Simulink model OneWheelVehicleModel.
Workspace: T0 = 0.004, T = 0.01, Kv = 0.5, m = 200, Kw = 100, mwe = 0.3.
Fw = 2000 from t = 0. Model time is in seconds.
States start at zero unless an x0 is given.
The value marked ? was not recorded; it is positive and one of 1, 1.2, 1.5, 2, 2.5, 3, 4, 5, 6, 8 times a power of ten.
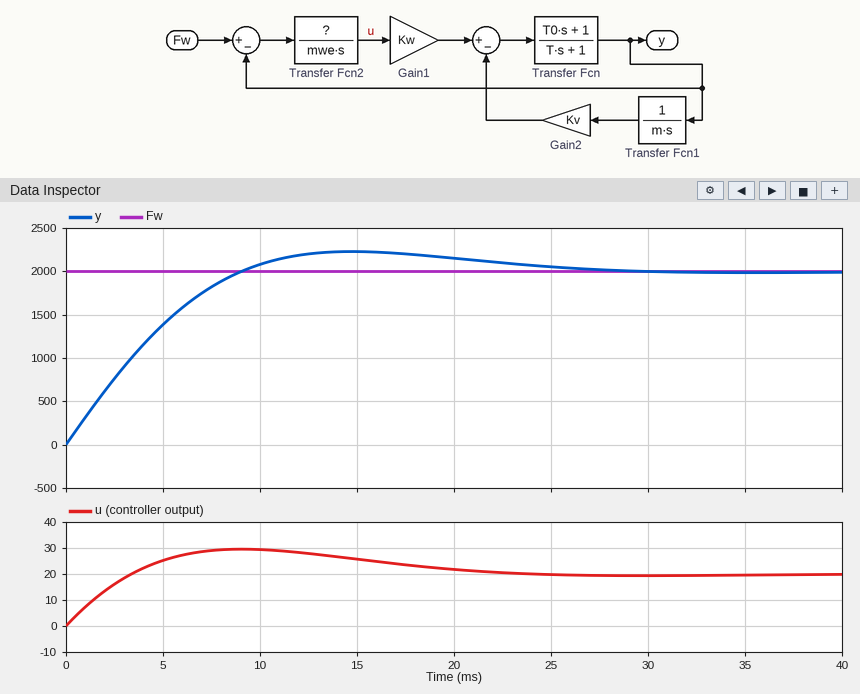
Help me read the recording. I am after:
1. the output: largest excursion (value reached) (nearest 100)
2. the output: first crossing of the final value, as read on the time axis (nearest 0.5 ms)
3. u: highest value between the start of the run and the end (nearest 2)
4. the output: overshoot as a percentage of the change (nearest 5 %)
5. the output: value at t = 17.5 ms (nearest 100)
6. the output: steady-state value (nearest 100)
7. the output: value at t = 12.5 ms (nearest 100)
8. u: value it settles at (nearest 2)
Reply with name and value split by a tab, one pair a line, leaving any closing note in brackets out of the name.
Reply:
the output: largest excursion (value reached)	2200
the output: first crossing of the final value, as read on the time axis	9.0 ms
u: highest value between the start of the run and the end	30
the output: overshoot as a percentage of the change	10 %
the output: value at t = 17.5 ms	2200
the output: steady-state value	2000
the output: value at t = 12.5 ms	2200
u: value it settles at	20
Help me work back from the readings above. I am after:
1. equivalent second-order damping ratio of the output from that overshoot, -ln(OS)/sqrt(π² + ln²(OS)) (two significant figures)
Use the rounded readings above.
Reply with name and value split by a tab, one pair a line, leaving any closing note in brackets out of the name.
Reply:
equivalent second-order damping ratio of the output from that overshoot, -ln(OS)/sqrt(π² + ln²(OS))	0.59
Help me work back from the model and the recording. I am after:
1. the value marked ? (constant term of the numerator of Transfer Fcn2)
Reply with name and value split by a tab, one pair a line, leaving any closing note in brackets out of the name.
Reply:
the value marked ?	1.2
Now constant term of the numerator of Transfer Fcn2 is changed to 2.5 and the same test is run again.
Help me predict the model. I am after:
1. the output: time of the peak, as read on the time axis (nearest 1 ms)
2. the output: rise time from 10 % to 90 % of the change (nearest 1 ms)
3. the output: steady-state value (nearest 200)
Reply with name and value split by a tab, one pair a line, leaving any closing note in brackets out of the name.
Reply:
the output: time of the peak, as read on the time axis	9 ms
the output: rise time from 10 % to 90 % of the change	4 ms
the output: steady-state value	2000
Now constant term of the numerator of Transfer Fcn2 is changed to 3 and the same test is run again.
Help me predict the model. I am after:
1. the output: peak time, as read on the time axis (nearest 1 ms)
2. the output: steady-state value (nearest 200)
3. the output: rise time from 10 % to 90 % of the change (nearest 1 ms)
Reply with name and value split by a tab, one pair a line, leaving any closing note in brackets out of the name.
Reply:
the output: peak time, as read on the time axis	8 ms
the output: steady-state value	2000
the output: rise time from 10 % to 90 % of the change	3 ms
